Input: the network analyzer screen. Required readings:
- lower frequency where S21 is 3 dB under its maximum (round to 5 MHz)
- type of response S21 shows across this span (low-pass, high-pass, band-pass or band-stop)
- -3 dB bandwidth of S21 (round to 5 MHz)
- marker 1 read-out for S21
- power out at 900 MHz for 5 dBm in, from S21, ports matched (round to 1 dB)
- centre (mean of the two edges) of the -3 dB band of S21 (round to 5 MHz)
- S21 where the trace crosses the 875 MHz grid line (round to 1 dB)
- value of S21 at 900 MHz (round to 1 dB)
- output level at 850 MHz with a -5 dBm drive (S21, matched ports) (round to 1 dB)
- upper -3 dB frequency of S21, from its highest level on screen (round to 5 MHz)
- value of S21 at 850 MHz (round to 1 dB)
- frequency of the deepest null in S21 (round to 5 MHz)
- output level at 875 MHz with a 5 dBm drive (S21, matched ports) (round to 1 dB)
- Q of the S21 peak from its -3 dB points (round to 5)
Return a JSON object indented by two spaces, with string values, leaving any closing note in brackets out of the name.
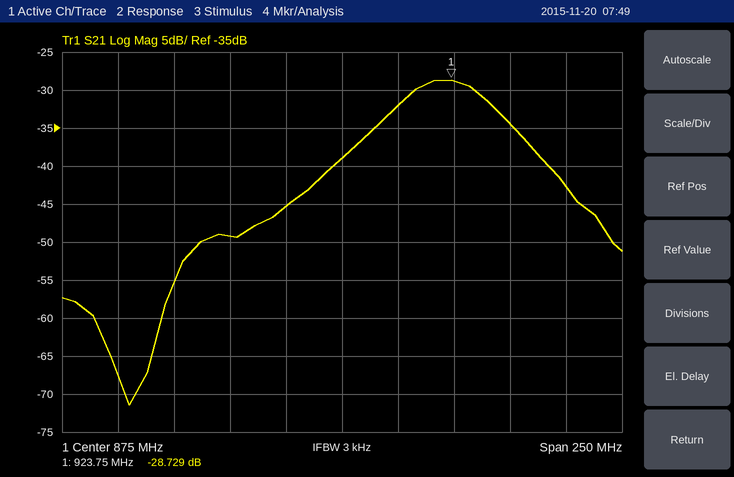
{
  "lower frequency where S21 is 3 dB under its maximum": "900 MHz",
  "type of response S21 shows across this span": "band-pass",
  "-3 dB bandwidth of S21": "40 MHz",
  "marker 1 read-out for S21": "-28.729 dB",
  "power out at 900 MHz for 5 dBm in, from S21, ports matched": "-27 dBm",
  "centre (mean of the two edges) of the -3 dB band of S21": "920 MHz",
  "S21 where the trace crosses the 875 MHz grid line": "-39 dB",
  "value of S21 at 900 MHz": "-32 dB",
  "output level at 850 MHz with a -5 dBm drive (S21, matched ports)": "-50 dBm",
  "upper -3 dB frequency of S21, from its highest level on screen": "940 MHz",
  "value of S21 at 850 MHz": "-45 dB",
  "frequency of the deepest null in S21": "780 MHz",
  "output level at 875 MHz with a 5 dBm drive (S21, matched ports)": "-34 dBm",
  "Q of the S21 peak from its -3 dB points": "25"
}
